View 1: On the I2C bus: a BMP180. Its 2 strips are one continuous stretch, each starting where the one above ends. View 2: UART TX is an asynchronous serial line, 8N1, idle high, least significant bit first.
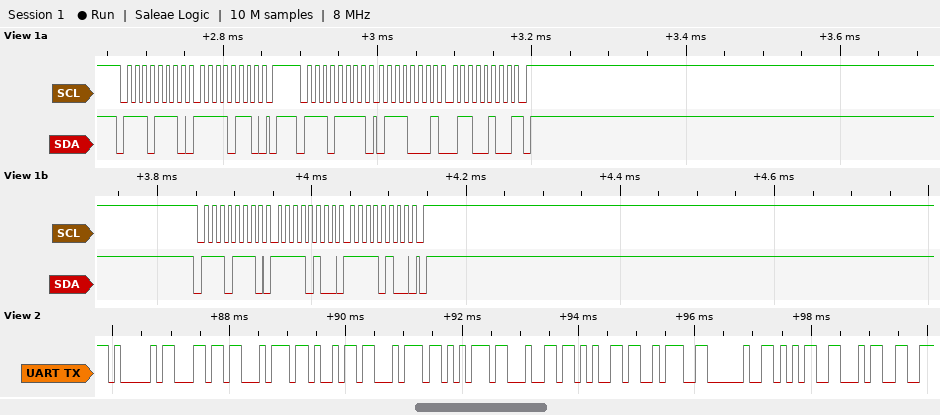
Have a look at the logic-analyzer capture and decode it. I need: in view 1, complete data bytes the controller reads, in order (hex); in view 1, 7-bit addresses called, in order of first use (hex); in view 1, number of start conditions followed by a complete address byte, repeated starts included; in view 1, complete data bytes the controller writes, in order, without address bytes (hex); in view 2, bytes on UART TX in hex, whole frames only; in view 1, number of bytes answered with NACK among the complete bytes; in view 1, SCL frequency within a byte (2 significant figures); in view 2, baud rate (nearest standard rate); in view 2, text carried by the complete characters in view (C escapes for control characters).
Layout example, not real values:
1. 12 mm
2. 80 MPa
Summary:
1. 71 64
2. 0x77
3. 3
4. F6 F4 F4
5. 41 6C 74 69 74 75 64 65 3A 20 35 34
6. 1
7. 100 kHz
8. 9600 baud
9. "Altitude: 54"
